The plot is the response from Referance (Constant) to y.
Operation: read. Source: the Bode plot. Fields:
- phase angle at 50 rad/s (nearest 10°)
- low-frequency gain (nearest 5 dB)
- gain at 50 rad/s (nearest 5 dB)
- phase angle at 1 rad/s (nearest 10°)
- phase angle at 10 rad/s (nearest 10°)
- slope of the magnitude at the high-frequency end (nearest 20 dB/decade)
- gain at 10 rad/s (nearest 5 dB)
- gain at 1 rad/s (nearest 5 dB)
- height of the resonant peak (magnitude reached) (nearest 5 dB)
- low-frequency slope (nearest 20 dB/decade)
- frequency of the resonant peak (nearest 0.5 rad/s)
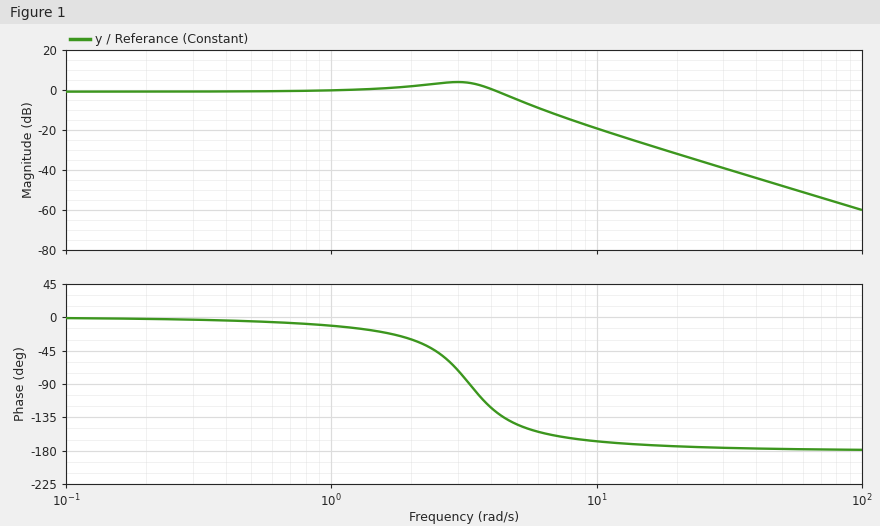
-180°
0 dB
-50 dB
-10°
-170°
-40 dB/decade
-20 dB
0 dB
5 dB
0 dB/decade
3.0 rad/s
